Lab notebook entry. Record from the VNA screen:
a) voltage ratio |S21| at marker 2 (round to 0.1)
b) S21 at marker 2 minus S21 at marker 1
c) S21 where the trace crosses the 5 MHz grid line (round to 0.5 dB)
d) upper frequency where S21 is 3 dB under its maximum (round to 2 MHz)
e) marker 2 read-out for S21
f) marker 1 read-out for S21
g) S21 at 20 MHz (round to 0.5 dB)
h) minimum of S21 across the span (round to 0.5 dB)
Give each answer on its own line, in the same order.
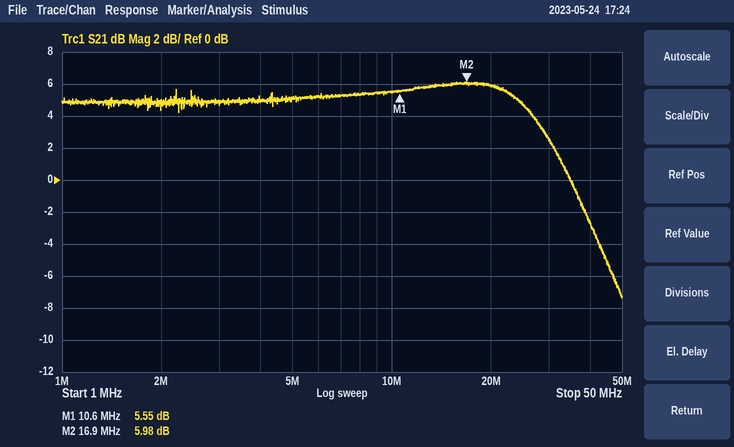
2.0
0.43 dB
5.0 dB
28 MHz
5.98 dB
5.55 dB
6.0 dB
-7.5 dB
